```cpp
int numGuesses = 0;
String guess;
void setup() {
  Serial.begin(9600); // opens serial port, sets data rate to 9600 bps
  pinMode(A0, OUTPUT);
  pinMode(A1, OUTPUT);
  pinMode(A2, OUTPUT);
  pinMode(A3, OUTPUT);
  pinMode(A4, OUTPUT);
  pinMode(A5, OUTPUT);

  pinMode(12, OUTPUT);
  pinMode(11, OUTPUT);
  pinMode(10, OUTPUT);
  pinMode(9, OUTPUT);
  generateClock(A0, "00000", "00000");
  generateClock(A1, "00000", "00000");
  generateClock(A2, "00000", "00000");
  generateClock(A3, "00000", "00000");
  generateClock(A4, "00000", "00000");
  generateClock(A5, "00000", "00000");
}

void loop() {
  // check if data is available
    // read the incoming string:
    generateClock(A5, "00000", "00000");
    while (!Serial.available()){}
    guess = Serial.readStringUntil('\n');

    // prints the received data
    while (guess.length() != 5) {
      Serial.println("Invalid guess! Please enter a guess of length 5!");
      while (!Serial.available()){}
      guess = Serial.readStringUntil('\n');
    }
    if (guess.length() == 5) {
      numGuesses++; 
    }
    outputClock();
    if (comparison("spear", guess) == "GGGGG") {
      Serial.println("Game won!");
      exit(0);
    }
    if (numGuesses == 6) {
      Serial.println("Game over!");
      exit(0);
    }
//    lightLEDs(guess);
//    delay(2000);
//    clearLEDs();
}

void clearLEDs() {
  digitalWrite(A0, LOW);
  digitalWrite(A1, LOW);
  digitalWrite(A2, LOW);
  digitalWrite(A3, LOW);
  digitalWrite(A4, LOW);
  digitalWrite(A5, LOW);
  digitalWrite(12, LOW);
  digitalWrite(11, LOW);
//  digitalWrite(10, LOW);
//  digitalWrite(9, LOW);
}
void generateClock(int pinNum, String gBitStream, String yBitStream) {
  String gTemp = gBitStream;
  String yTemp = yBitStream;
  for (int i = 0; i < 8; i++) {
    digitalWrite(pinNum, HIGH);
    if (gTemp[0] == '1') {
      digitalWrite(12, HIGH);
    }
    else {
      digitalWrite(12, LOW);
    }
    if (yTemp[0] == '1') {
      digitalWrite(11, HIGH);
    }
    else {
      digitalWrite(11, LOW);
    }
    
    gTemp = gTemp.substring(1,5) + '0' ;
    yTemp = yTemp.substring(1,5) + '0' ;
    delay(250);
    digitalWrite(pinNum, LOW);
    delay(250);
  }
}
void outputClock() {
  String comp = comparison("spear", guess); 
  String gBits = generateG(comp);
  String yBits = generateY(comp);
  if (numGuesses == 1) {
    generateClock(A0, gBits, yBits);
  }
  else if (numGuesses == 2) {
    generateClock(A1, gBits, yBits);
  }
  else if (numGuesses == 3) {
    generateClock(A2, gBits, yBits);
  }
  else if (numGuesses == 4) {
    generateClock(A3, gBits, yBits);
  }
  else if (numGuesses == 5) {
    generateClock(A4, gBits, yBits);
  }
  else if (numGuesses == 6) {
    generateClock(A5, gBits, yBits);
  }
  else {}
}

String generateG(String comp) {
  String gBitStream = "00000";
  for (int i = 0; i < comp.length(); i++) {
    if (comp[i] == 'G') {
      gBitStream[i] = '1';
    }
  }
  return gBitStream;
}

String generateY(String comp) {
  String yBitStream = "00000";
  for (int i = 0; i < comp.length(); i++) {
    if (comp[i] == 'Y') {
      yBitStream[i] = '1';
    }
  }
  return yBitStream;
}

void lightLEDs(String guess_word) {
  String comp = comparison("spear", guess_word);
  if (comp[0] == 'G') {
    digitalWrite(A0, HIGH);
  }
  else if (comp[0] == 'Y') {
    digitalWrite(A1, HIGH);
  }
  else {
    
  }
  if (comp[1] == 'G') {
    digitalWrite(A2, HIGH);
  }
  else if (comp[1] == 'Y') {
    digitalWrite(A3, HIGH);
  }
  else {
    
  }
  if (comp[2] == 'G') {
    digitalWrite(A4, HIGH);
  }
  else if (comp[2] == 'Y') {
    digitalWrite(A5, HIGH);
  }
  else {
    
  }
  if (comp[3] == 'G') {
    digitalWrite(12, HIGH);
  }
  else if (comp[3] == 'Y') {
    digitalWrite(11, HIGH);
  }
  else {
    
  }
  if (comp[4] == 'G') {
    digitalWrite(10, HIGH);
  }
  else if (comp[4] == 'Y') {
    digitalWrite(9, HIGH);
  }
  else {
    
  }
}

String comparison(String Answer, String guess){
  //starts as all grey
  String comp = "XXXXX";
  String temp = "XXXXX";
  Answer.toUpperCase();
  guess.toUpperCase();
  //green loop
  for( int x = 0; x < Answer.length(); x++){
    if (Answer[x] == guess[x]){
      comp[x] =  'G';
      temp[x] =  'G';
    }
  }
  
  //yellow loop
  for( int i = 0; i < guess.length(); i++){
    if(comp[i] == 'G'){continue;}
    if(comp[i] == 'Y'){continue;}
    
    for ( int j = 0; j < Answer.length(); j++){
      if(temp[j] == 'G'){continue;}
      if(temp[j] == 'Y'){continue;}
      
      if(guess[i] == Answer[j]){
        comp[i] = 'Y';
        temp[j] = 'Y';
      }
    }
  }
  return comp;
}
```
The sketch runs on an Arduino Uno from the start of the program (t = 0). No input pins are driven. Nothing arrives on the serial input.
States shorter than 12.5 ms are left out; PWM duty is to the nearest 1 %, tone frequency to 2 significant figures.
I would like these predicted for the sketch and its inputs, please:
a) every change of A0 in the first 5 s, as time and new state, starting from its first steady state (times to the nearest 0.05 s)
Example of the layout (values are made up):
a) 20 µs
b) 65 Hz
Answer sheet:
a) 0 s high; 0.25 s low; 0.5 s high; 0.75 s low; 1 s high; 1.25 s low; 1.5 s high; 1.75 s low; 2 s high; 2.25 s low; 2.5 s high; 2.75 s low; 3 s high; 3.25 s low; 3.5 s high; 3.75 s low
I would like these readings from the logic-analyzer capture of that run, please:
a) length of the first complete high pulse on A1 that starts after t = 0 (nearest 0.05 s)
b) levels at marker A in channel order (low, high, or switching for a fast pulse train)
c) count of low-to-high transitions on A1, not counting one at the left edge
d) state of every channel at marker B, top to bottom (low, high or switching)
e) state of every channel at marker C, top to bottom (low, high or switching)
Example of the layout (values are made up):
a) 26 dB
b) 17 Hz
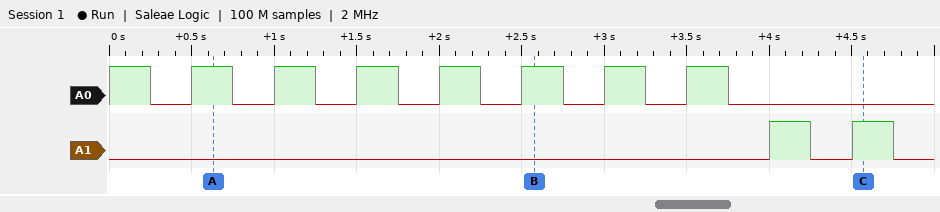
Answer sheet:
a) 0.25 s
b) A0 high, A1 low
c) 2
d) A0 high, A1 low
e) A0 low, A1 high
